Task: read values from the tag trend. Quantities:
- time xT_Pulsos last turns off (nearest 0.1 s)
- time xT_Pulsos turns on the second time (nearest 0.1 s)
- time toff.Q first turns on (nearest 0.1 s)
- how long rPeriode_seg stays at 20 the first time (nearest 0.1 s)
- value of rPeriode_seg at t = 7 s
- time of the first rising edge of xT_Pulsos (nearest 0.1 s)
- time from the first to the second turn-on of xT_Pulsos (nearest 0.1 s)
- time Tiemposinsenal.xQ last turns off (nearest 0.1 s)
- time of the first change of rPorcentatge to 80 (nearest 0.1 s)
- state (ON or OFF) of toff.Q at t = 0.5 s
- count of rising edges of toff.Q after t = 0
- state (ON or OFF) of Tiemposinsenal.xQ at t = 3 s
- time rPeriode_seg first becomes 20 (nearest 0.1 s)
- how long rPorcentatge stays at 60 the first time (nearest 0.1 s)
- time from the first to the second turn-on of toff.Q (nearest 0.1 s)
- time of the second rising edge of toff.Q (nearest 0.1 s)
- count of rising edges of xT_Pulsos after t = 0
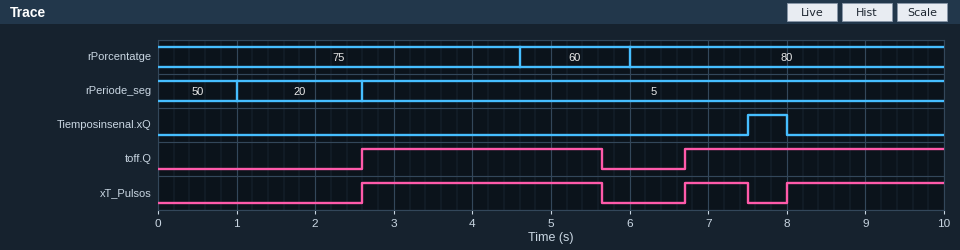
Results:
7.5 s
6.7 s
2.6 s
1.6 s
5
2.6 s
4.1 s
8.0 s
6.0 s
OFF
2
OFF
1.0 s
1.4 s
4.1 s
6.7 s
3
